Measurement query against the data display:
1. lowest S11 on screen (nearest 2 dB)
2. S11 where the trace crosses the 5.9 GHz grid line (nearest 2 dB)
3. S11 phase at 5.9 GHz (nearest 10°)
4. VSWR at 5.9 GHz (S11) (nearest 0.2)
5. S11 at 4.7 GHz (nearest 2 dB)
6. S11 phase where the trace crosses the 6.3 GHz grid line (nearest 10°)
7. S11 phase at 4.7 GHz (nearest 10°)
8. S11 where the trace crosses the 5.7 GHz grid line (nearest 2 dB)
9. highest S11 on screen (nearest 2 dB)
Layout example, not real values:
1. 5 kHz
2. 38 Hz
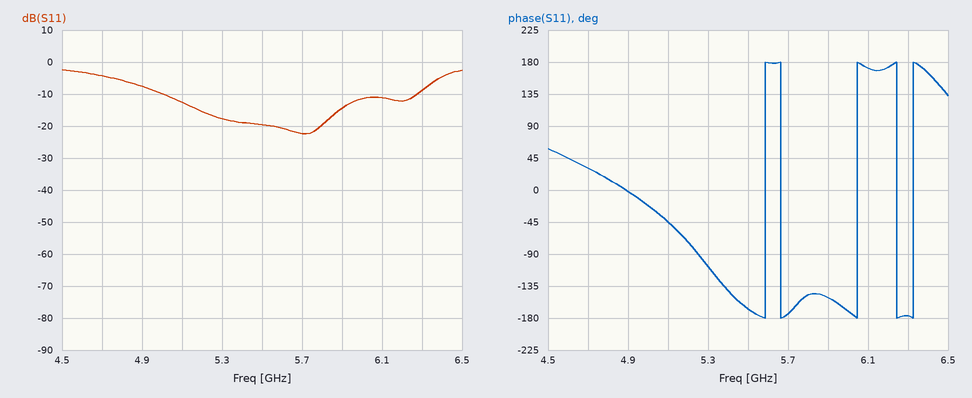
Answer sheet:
1. -22 dB
2. -14 dB
3. -150°
4. 1.4
5. -4 dB
6. -180°
7. 30°
8. -22 dB
9. -2 dB
